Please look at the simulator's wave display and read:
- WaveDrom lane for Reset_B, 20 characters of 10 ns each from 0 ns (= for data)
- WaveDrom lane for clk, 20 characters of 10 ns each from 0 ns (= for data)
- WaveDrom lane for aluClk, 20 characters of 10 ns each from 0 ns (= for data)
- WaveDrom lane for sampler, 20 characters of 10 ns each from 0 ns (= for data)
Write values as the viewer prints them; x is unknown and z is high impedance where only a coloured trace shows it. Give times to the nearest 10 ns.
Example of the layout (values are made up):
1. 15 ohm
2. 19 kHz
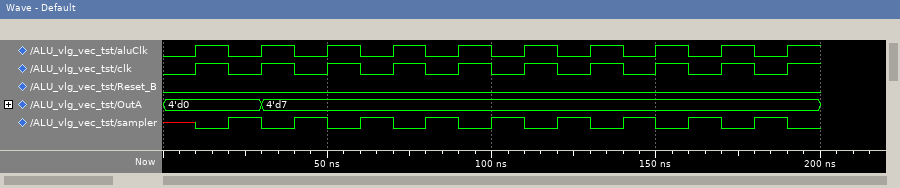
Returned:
1. {name: 'Reset_B', wave: '0...................'}
2. {name: 'clk', wave: '01010101010101010101'}
3. {name: 'aluClk', wave: '01010101010101010101'}
4. {name: 'sampler', wave: 'x0101010101010101010'}
